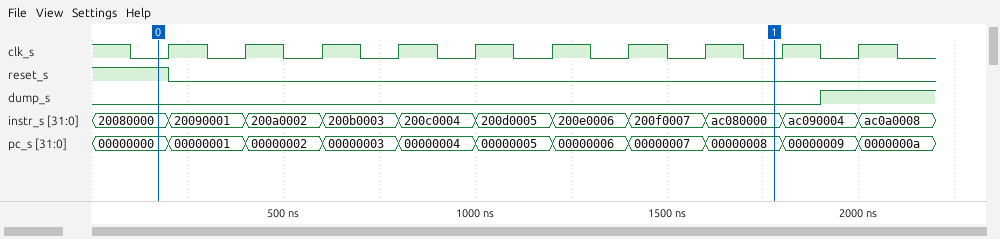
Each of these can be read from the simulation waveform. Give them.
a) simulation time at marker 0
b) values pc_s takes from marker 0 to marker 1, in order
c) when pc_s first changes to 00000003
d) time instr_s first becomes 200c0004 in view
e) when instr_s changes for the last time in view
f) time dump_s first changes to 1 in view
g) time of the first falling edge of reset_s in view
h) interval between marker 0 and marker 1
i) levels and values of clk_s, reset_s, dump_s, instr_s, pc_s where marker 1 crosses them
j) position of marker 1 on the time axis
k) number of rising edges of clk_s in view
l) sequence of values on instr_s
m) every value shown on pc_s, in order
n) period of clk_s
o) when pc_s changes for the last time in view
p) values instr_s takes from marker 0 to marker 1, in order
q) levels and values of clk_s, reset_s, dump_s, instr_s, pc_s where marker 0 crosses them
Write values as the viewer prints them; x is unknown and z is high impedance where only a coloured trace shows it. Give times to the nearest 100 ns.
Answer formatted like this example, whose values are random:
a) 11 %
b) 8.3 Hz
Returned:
a) 200 ns
b) 00000000, 00000001, 00000002, 00000003, 00000004, 00000005, 00000006, 00000007, 00000008
c) 600 ns
d) 800 ns
e) 2000 ns
f) 1900 ns
g) 200 ns
h) 1600 ns
i) clk_s=0, reset_s=0, dump_s=0, instr_s=ac080000, pc_s=00000008
j) 1800 ns
k) 10
l) 20080000, 20090001, 200a0002, 200b0003, 200c0004, 200d0005, 200e0006, 200f0007, ac080000, ac090004, ac0a0008
m) 00000000, 00000001, 00000002, 00000003, 00000004, 00000005, 00000006, 00000007, 00000008, 00000009, 0000000a
n) 200 ns
o) 2000 ns
p) 20080000, 20090001, 200a0002, 200b0003, 200c0004, 200d0005, 200e0006, 200f0007, ac080000
q) clk_s=0, reset_s=1, dump_s=0, instr_s=20080000, pc_s=00000000
